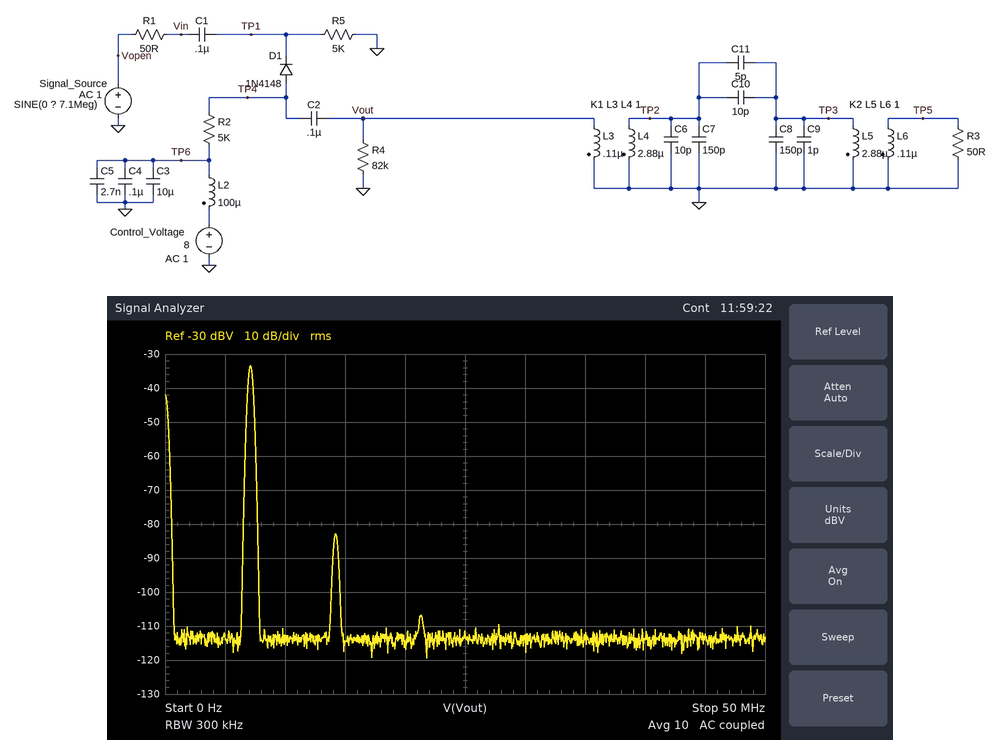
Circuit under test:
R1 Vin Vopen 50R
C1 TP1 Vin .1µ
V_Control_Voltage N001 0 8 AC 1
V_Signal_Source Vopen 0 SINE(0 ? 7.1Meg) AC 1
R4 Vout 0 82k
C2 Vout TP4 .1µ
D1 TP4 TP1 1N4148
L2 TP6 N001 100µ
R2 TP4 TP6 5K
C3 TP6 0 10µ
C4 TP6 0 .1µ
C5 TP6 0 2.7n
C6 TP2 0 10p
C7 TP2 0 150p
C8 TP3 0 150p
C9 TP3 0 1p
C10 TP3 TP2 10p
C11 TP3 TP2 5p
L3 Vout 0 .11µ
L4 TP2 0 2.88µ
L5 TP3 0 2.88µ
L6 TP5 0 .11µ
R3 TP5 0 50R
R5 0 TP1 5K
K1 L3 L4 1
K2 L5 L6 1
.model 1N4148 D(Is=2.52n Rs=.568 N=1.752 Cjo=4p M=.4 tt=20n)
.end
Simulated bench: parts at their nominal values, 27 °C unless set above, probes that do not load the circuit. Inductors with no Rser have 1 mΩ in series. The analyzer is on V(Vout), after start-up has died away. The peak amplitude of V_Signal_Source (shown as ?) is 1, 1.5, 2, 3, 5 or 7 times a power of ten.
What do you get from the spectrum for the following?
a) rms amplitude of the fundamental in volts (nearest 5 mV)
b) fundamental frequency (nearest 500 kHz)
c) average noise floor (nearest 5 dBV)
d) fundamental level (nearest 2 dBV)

20 mV
7.0 MHz
-115 dBV
-34 dBV
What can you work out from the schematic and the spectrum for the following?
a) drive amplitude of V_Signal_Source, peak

70 mV
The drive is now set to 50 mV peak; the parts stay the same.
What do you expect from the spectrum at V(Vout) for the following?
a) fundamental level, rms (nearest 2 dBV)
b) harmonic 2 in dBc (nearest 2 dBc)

-36 dBV
-52 dBc
